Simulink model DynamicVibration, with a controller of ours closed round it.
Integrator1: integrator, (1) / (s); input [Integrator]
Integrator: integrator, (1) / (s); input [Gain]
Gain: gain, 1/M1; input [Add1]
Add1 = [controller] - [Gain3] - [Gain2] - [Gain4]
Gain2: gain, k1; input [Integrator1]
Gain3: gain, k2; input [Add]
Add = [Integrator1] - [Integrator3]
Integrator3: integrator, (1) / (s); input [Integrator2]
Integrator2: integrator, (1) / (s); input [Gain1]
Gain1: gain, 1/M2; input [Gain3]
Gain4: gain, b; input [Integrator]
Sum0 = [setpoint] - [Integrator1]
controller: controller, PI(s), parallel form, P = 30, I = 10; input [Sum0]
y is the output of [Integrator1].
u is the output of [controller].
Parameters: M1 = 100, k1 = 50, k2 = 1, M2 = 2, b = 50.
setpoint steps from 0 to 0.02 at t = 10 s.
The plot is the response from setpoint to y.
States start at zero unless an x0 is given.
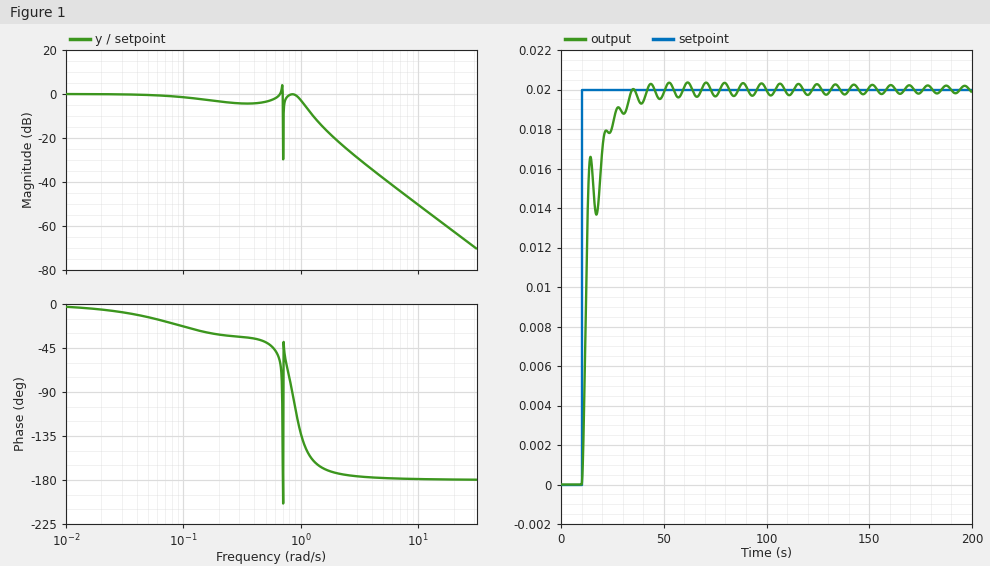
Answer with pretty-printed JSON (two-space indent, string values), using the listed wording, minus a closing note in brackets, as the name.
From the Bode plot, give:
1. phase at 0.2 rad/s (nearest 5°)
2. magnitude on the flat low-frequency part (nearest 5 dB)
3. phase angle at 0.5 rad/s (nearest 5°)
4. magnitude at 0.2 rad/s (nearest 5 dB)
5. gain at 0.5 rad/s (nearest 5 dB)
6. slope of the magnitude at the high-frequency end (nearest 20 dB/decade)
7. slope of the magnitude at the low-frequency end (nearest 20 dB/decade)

{
  "phase at 0.2 rad/s": "-30°",
  "magnitude on the flat low-frequency part": "0 dB",
  "phase angle at 0.5 rad/s": "-40°",
  "magnitude at 0.2 rad/s": "-5 dB",
  "gain at 0.5 rad/s": "-5 dB",
  "slope of the magnitude at the high-frequency end": "-40 dB/decade",
  "slope of the magnitude at the low-frequency end": "0 dB/decade"
}
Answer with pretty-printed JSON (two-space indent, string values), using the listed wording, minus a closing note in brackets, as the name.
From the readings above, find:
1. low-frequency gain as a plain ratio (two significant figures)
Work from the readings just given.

{
  "low-frequency gain as a plain ratio": "1.0"
}
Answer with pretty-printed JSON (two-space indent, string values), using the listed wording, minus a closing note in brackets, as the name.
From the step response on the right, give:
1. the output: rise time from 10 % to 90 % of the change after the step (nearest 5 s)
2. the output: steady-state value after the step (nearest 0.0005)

{
  "the output: rise time from 10 % to 90 % of the change after the step": "15 s",
  "the output: steady-state value after the step": "0.0200"
}
